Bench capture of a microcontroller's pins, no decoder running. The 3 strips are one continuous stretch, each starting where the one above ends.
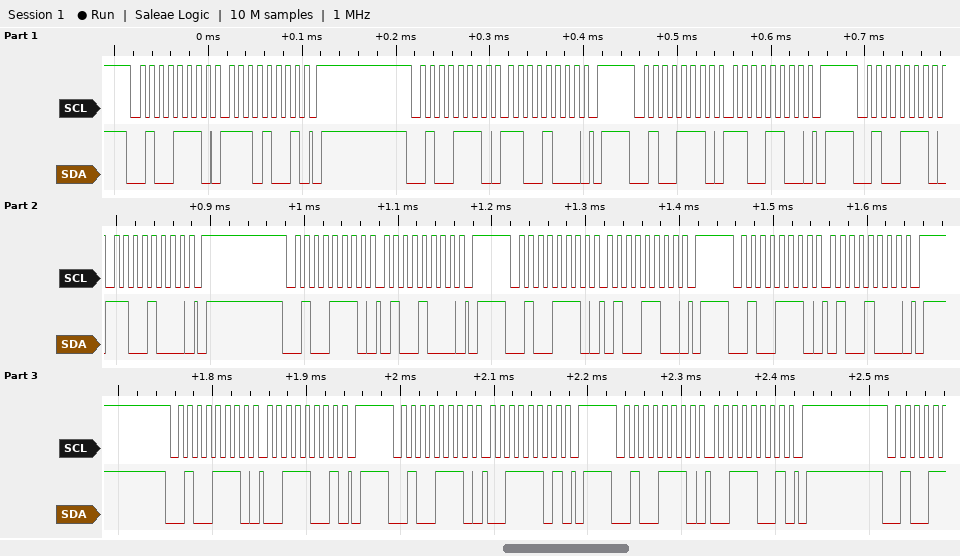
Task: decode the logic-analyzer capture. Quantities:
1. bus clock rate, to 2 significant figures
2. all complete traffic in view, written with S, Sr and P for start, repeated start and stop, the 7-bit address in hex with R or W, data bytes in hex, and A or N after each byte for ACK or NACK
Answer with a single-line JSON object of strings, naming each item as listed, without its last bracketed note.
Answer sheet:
{"bus clock rate, to 2 significant figures": "100 kHz", "all complete traffic in view, written with S, Sr and P for start, repeated start and stop, the 7-bit address in hex with R or W, data bytes in hex, and A or N after each byte for ACK or NACK": "S 27W A E9 A P S 27W A C8 A P S 27W A CC A P S 27W A C8 A P S 27W A 48 A P S 27W A 4C A P S 27W A 48 A P S 27W A 39 A P S 27W A 3D A P S 27W A 39 A P"}
